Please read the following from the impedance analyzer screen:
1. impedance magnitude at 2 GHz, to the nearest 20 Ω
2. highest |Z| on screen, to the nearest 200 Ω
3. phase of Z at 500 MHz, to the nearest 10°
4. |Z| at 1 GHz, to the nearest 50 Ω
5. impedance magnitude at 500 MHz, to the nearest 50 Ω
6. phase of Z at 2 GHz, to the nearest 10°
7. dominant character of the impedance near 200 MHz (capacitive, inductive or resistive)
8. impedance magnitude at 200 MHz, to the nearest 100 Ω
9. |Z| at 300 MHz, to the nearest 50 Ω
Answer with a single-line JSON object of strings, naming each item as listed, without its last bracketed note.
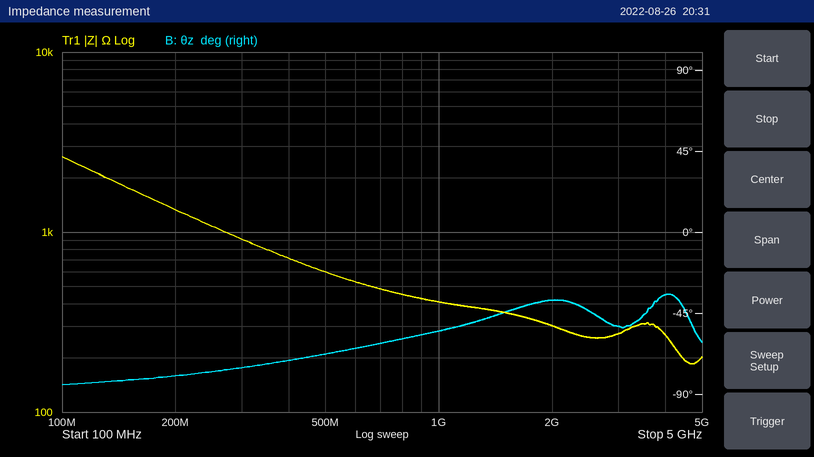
{"impedance magnitude at 2 GHz, to the nearest 20 Ω": "300 Ω", "highest |Z| on screen, to the nearest 200 Ω": "2.6 kΩ", "phase of Z at 500 MHz, to the nearest 10°": "-70°", "|Z| at 1 GHz, to the nearest 50 Ω": "400 Ω", "impedance magnitude at 500 MHz, to the nearest 50 Ω": "600 Ω", "phase of Z at 2 GHz, to the nearest 10°": "-40°", "dominant character of the impedance near 200 MHz": "capacitive", "impedance magnitude at 200 MHz, to the nearest 100 Ω": "1.3 kΩ", "|Z| at 300 MHz, to the nearest 50 Ω": "900 Ω"}
